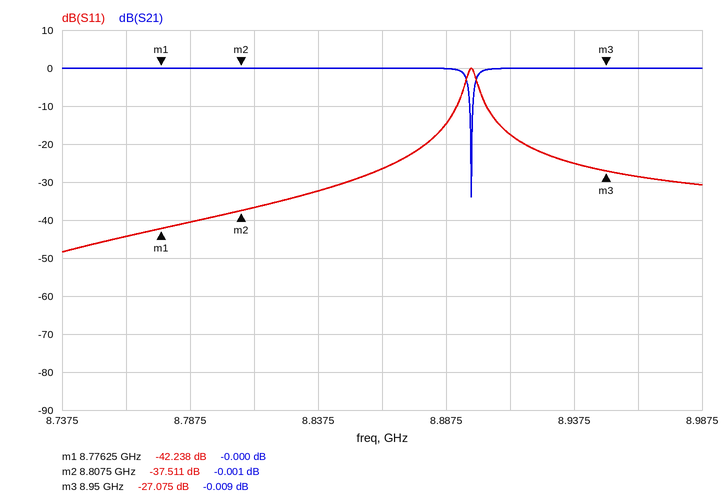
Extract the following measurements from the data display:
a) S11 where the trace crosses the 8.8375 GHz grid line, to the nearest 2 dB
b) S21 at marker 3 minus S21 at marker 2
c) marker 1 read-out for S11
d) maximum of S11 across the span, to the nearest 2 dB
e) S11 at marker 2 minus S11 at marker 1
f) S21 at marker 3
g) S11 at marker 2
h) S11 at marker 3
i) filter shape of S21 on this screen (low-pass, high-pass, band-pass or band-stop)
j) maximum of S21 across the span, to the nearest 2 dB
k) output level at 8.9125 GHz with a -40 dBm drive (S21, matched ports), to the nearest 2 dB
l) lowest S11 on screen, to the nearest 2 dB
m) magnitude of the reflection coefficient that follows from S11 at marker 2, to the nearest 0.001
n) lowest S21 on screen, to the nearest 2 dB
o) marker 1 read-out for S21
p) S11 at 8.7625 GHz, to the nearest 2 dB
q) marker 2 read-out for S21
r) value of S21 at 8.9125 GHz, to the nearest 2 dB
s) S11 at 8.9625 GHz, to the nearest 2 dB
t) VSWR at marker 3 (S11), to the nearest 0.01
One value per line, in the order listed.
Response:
-32 dB
-0.008 dB
-42.238 dB
0 dB
4.727 dB
-0.009 dB
-37.511 dB
-27.075 dB
band-stop
0 dB
-40 dBm
-48 dB
0.013
-34 dB
-0.000 dB
-44 dB
-0.001 dB
0 dB
-28 dB
1.09
